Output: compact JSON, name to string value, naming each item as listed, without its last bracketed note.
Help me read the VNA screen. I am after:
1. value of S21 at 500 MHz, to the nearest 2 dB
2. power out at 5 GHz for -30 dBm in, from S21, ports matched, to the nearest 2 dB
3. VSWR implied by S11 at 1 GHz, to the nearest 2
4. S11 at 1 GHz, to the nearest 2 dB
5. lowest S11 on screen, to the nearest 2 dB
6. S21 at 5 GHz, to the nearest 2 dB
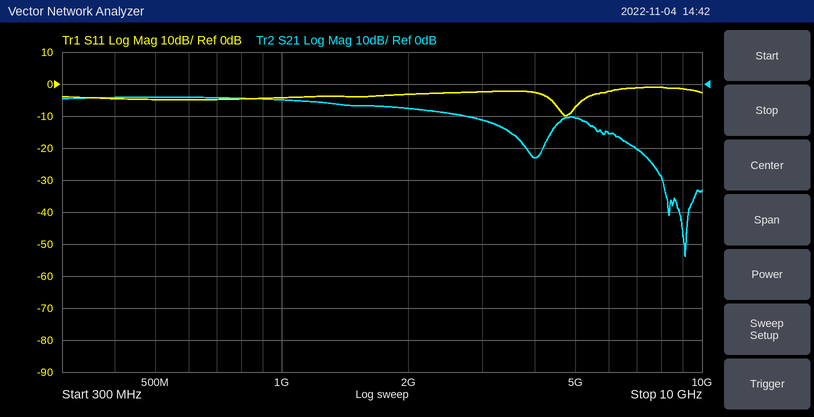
{"value of S21 at 500 MHz, to the nearest 2 dB": "-4 dB", "power out at 5 GHz for -30 dBm in, from S21, ports matched, to the nearest 2 dB": "-40 dBm", "VSWR implied by S11 at 1 GHz, to the nearest 2": "4", "S11 at 1 GHz, to the nearest 2 dB": "-4 dB", "lowest S11 on screen, to the nearest 2 dB": "-10 dB", "S21 at 5 GHz, to the nearest 2 dB": "-10 dB"}
